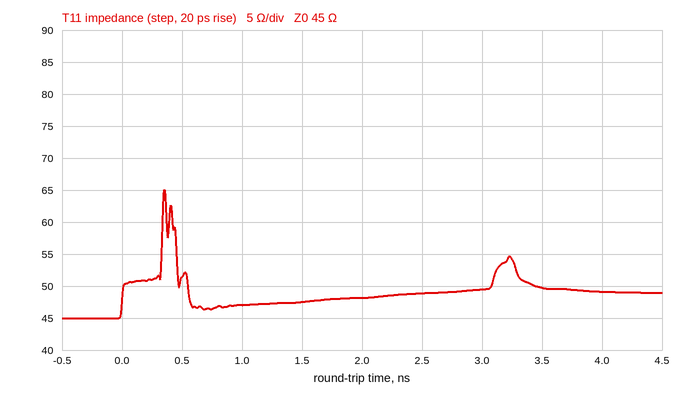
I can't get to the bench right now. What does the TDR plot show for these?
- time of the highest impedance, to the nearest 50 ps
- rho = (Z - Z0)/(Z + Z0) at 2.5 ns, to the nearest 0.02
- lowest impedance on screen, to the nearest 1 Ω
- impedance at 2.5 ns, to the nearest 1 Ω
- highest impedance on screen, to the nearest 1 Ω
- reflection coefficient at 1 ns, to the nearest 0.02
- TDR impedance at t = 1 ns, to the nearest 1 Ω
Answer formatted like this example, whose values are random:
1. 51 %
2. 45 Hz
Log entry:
1. 350 ps
2. +0.04
3. 45 Ω
4. 49 Ω
5. 65 Ω
6. +0.02
7. 47 Ω
